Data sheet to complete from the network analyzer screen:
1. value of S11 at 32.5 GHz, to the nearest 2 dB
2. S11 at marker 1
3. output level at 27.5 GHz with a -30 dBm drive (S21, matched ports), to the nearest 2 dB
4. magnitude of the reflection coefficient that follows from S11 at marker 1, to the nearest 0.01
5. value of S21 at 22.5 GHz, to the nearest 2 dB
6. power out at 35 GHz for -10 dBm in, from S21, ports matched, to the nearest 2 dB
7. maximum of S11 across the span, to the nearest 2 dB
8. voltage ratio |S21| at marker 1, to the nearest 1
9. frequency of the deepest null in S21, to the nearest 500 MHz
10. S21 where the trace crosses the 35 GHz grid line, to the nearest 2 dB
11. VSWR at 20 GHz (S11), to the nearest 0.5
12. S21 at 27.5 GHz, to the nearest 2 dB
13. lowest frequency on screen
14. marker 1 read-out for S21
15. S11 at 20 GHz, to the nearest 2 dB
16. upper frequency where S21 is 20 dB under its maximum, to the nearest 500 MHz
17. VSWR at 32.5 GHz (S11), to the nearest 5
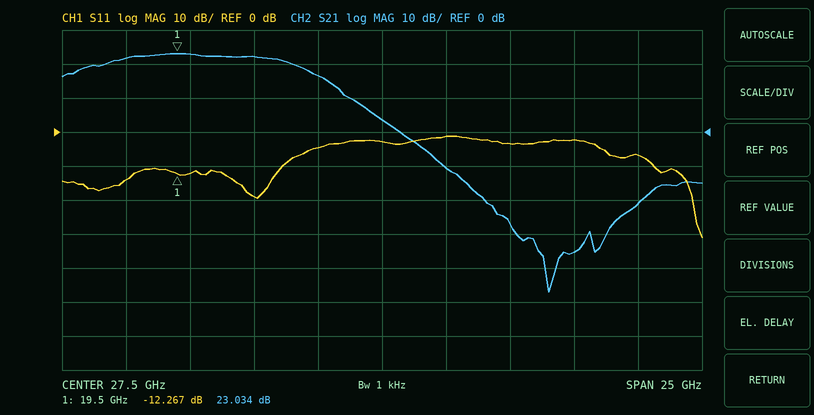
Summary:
-4 dB
-12.267 dB
-26 dBm
0.24
22 dB
-46 dBm
-2 dB
14
34.0 GHz
-36 dB
1.5
4 dB
15 GHz
23.034 dB
-12 dB
27.5 GHz
5
